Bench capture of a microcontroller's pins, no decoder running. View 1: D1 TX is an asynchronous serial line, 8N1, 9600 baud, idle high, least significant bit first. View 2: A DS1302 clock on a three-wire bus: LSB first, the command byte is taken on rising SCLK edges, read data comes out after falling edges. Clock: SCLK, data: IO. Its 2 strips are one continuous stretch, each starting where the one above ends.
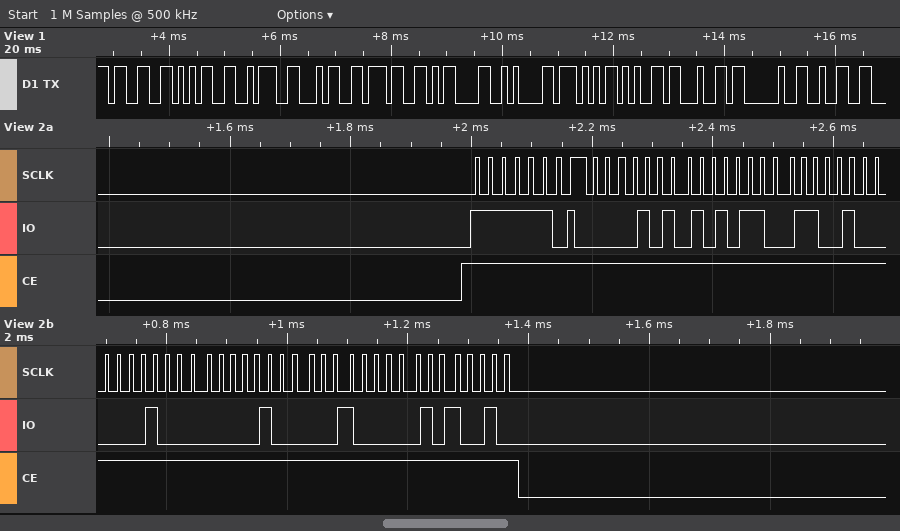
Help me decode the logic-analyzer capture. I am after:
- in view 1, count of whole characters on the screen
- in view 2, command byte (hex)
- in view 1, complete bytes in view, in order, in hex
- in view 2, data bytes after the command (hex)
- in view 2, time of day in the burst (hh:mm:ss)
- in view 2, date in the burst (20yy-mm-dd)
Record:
12
0xBF
33 35 3A 34 37 0D 0A 57 65 64 20 32
50 35 13 08 10 04 25
13:35:50
2025-10-08
